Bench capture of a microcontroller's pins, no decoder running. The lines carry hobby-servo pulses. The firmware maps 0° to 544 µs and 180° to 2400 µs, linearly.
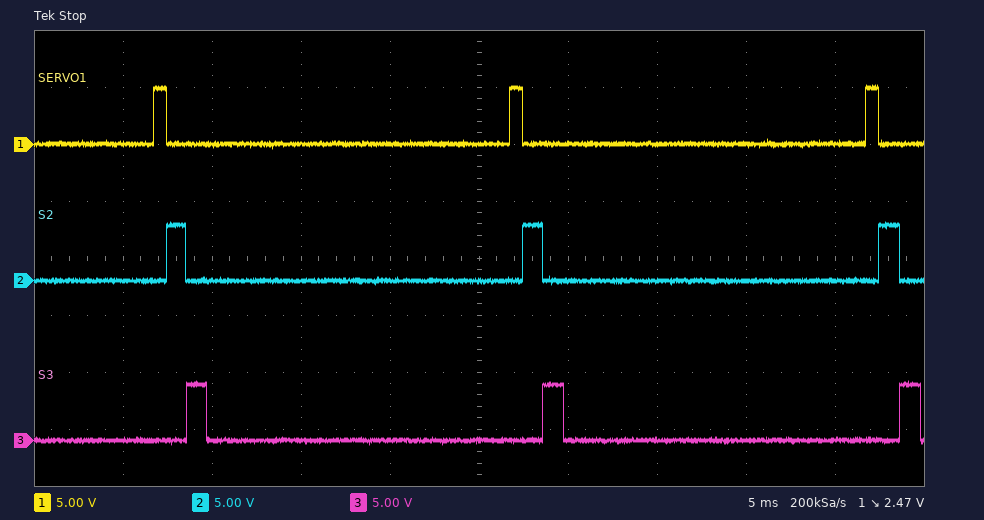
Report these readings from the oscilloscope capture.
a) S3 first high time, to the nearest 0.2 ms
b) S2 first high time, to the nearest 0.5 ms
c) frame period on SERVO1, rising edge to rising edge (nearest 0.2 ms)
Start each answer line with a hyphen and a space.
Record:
- 1.2 ms
- 1.0 ms
- 20.0 ms
